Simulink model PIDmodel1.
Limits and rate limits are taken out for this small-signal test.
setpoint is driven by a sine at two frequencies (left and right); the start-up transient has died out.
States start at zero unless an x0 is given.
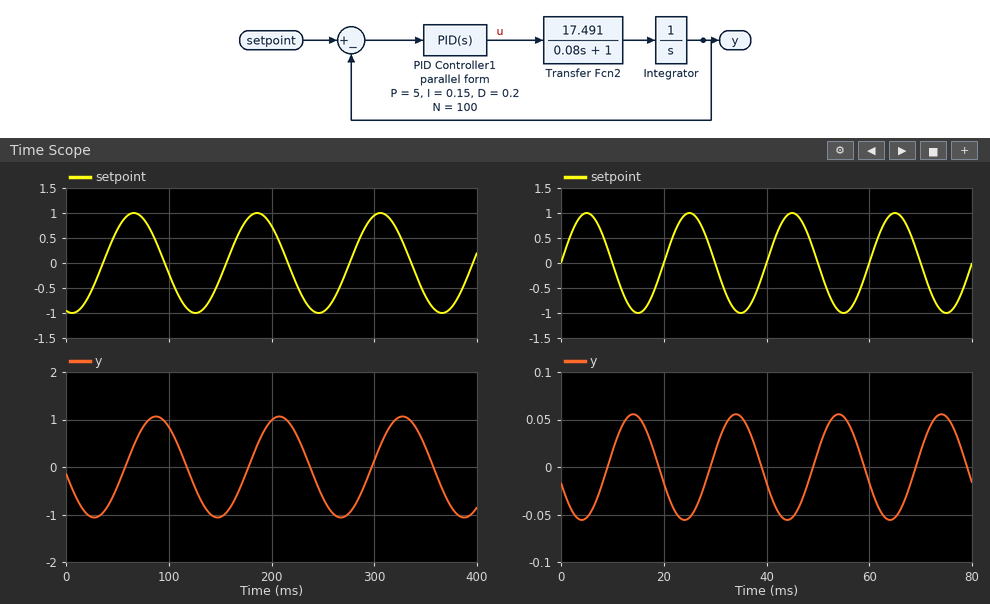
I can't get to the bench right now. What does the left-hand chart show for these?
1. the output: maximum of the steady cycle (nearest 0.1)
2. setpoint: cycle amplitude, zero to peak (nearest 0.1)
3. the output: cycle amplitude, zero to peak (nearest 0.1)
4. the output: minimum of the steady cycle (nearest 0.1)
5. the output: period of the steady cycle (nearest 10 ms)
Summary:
1.1
1.0
1.1
-1.1
120 ms
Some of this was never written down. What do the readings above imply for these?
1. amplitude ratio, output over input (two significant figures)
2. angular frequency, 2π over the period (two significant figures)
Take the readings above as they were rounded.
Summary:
1.1
0.052 rad/ms
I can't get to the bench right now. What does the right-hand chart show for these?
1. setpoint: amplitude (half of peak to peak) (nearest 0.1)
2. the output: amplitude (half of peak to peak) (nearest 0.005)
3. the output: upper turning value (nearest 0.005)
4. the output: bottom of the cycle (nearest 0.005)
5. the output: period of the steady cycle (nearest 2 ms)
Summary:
1.0
0.055
0.055
-0.055
20 ms
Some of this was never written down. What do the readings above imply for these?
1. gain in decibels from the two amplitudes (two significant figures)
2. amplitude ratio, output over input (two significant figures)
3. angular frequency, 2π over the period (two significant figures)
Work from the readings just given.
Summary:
-25 dB
0.055
0.31 rad/ms
